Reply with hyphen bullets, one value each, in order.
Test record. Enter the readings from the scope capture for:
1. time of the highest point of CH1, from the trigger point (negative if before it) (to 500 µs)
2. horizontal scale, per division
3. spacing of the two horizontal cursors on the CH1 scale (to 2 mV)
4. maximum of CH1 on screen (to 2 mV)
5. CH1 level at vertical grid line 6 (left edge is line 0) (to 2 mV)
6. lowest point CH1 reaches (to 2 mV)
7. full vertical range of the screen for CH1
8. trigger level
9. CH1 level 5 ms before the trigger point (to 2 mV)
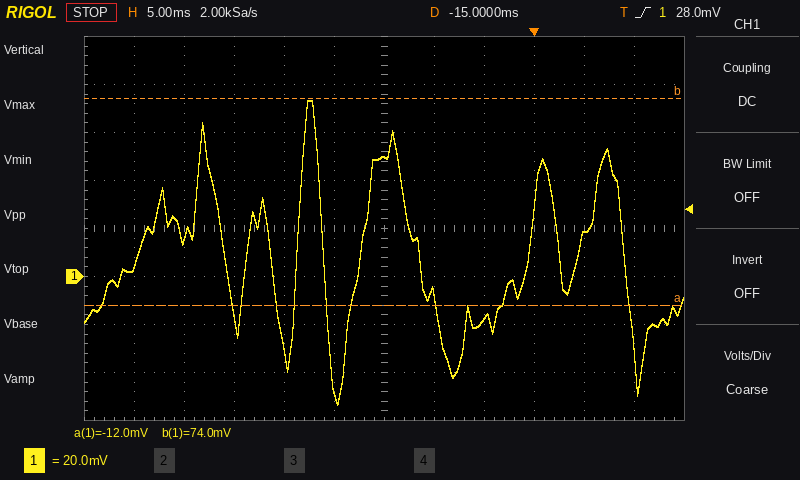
- -22.5 ms
- 5 ms
- 86 mV
- 74 mV
- 50 mV
- -54 mV
- 160 mV
- 28.0 mV
- -18 mV
